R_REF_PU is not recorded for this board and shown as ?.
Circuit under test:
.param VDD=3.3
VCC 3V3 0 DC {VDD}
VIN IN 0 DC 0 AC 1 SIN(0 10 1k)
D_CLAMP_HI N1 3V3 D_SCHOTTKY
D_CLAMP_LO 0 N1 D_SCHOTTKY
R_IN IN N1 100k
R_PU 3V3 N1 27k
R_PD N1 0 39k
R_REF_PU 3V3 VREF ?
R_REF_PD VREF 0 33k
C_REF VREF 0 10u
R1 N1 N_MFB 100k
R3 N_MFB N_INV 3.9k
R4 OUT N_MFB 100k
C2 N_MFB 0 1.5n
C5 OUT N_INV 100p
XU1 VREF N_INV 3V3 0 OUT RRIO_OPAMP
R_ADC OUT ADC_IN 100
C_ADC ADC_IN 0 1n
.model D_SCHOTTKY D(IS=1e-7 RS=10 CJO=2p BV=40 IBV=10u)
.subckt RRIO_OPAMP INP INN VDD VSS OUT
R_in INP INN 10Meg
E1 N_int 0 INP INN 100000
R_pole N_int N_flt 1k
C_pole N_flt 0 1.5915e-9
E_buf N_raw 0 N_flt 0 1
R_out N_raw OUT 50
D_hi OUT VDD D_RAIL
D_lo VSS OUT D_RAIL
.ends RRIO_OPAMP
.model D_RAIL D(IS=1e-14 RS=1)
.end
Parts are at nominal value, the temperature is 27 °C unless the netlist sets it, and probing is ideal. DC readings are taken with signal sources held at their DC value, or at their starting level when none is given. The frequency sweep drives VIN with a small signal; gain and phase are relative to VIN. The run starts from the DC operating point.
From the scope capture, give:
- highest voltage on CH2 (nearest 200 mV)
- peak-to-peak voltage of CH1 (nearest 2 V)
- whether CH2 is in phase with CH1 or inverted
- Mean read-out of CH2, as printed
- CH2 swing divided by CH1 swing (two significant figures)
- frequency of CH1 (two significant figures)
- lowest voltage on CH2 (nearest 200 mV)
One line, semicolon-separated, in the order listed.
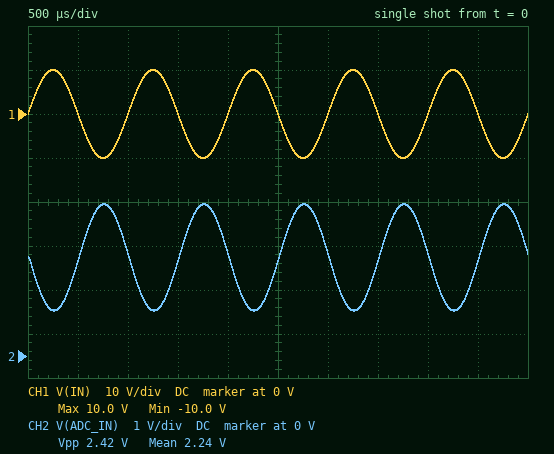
3.4 V; 20 V; inverted; 2.24 V; 0.12; 1.0 kHz; 1.0 V
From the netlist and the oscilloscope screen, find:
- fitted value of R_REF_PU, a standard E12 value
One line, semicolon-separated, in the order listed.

22 kΩ
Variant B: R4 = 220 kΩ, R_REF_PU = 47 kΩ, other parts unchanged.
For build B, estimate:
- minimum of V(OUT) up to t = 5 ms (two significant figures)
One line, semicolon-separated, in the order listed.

-1.9 V
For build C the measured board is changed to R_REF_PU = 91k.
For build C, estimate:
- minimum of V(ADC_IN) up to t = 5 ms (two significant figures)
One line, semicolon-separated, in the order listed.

-1.0 V
